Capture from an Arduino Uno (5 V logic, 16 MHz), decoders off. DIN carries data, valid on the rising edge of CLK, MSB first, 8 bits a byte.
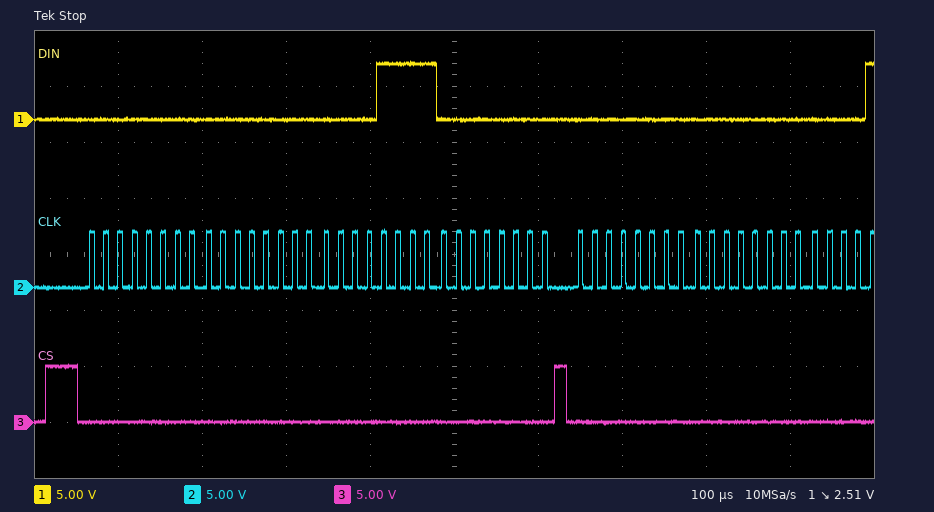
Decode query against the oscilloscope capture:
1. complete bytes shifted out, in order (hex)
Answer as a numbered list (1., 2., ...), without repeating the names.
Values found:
1. 00 00 0F 00 00 00
